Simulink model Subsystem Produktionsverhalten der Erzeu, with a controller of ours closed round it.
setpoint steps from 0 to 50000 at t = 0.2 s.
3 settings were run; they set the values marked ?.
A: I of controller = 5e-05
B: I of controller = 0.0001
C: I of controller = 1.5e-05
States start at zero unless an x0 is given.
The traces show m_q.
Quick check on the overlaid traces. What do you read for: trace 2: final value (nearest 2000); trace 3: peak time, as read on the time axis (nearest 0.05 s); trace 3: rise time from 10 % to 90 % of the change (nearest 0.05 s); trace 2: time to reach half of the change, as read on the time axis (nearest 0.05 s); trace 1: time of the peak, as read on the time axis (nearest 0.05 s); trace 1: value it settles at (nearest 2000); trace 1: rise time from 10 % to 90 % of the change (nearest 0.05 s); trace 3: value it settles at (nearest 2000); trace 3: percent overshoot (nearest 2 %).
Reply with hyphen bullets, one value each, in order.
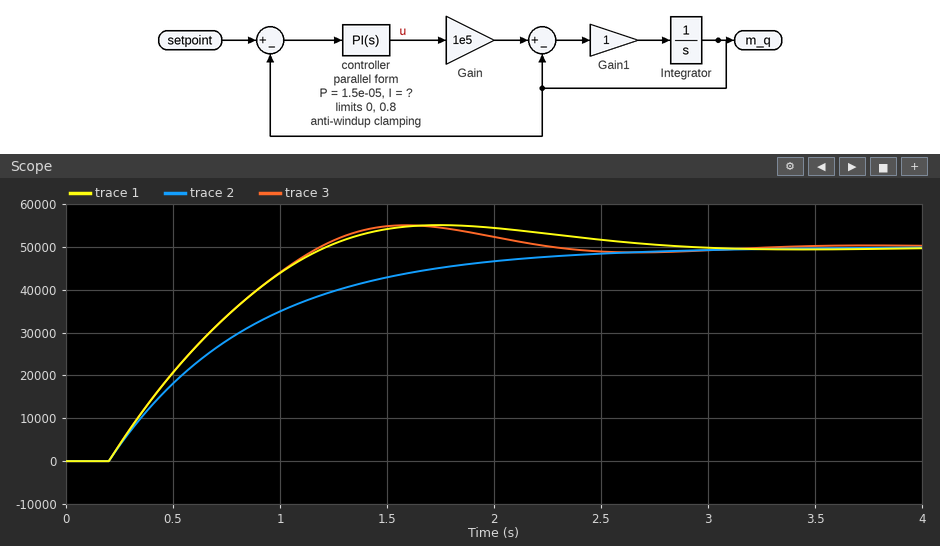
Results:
- 50000
- 1.60 s
- 0.75 s
- 0.65 s
- 1.75 s
- 50000
- 0.75 s
- 50000
- 10 %
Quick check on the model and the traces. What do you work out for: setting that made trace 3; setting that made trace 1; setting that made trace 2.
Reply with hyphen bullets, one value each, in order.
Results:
- B
- A
- C
